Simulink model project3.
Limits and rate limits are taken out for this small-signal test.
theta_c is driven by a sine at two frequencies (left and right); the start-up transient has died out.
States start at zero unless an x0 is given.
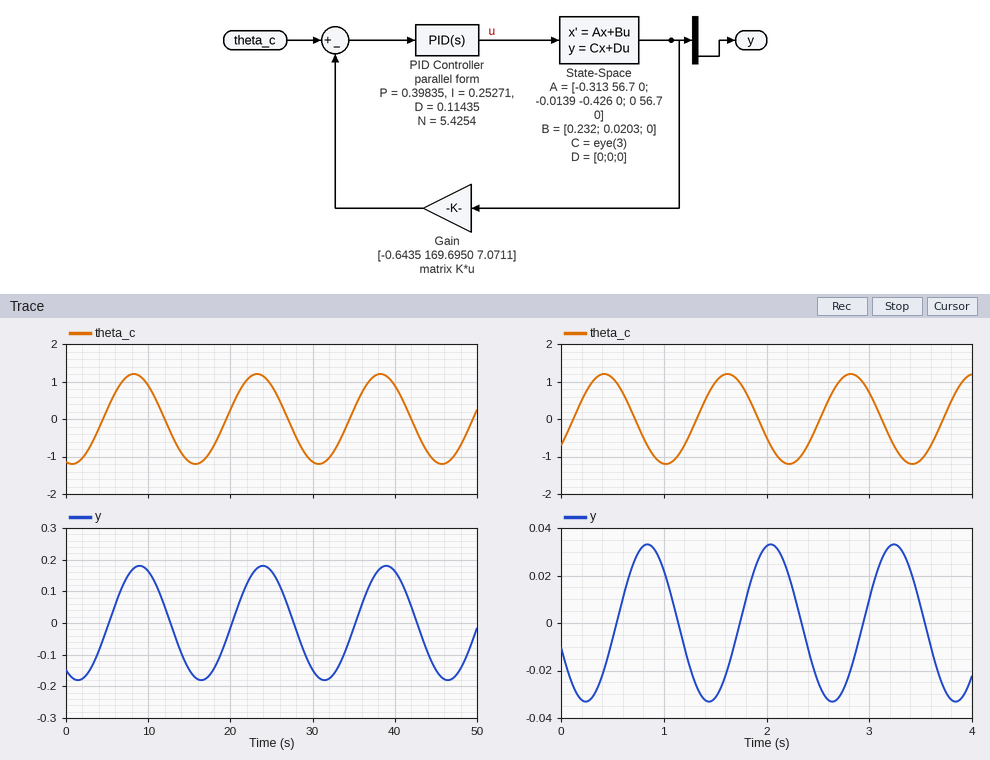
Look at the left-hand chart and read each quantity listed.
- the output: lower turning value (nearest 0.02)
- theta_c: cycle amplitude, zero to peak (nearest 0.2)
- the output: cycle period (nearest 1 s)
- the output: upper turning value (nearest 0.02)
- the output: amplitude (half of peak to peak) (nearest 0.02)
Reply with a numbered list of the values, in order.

1. -0.18
2. 1.2
3. 15 s
4. 0.18
5. 0.18
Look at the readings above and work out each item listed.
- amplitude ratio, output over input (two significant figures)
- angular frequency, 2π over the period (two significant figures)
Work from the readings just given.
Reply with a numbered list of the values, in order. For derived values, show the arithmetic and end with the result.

1. 0.18 / 1.2 = 0.15
2. 2π / 15 = 0.42 rad/s
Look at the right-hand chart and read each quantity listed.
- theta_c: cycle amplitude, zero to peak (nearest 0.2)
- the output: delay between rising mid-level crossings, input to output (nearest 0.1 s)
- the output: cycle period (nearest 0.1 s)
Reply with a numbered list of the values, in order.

1. 1.2
2. 0.4 s
3. 1.2 s
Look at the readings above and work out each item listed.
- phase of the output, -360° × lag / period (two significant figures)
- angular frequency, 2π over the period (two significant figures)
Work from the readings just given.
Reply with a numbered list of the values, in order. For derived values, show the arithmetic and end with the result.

1. -360 × 0.4 / 1.2 = -120°
2. 2π / 1.2 = 5.2 rad/s
